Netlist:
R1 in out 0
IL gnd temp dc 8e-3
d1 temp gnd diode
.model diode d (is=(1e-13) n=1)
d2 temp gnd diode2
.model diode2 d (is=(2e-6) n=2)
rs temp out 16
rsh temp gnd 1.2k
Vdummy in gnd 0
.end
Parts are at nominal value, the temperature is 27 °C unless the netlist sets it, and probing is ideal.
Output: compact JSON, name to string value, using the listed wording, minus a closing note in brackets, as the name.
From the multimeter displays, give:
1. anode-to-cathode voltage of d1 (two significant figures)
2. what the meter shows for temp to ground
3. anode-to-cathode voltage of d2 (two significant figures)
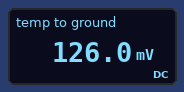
{"anode-to-cathode voltage of d1": "130 mV", "what the meter shows for temp to ground": "126.0 mV", "anode-to-cathode voltage of d2": "130 mV"}
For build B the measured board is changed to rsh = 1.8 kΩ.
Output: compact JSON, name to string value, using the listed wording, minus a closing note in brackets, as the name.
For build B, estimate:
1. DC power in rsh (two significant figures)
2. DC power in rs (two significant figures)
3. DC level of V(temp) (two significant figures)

{"DC power in rsh": "8.9 µW", "DC power in rs": "1.0 mW", "DC level of V(temp)": "130 mV"}
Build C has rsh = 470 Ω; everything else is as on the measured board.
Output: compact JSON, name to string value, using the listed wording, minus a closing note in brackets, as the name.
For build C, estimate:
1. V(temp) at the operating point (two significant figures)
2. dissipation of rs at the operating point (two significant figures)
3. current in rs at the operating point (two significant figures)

{"V(temp) at the operating point": "120 mV", "dissipation of rs at the operating point": "950 µW", "current in rs at the operating point": "7.7 mA"}
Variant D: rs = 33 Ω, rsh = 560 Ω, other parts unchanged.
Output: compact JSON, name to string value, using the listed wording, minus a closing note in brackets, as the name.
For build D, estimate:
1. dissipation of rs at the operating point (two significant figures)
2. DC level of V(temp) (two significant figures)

{"dissipation of rs at the operating point": "1.8 mW", "DC level of V(temp)": "240 mV"}
